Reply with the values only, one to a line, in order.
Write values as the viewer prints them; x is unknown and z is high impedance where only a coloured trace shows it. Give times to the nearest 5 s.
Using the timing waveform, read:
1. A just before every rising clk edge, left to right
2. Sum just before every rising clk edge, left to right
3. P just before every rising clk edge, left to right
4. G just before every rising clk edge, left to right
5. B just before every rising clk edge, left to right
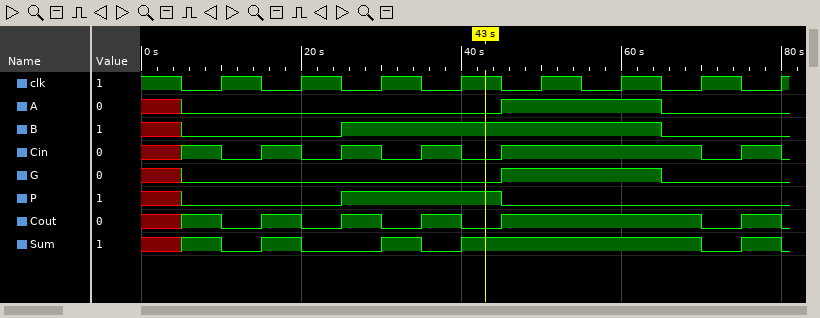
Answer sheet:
0 0 0 0 1 1 0 0
1 1 0 0 1 1 1 1
0 0 1 1 0 0 0 0
0 0 0 0 1 1 0 0
0 0 1 1 1 1 0 0
